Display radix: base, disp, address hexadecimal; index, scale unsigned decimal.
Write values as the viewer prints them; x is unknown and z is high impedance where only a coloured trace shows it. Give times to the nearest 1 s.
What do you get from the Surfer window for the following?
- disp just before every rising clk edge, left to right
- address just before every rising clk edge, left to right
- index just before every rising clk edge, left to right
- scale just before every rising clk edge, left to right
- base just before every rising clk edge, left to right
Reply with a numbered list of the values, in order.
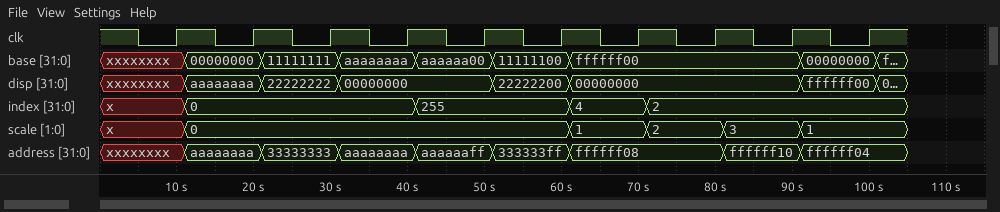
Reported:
1. xxxxxxxx, aaaaaaaa, 22222222, 00000000, 00000000, 22222200, 00000000, 00000000, 00000000, ffffff00
2. xxxxxxxx, aaaaaaaa, 33333333, aaaaaaaa, aaaaaaff, 333333ff, ffffff08, ffffff08, ffffff10, ffffff04
3. x, 0, 0, 0, 255, 255, 4, 2, 2, 2
4. x, 0, 0, 0, 0, 0, 1, 2, 3, 1
5. xxxxxxxx, 00000000, 11111111, aaaaaaaa, aaaaaa00, 11111100, ffffff00, ffffff00, ffffff00, 00000000
